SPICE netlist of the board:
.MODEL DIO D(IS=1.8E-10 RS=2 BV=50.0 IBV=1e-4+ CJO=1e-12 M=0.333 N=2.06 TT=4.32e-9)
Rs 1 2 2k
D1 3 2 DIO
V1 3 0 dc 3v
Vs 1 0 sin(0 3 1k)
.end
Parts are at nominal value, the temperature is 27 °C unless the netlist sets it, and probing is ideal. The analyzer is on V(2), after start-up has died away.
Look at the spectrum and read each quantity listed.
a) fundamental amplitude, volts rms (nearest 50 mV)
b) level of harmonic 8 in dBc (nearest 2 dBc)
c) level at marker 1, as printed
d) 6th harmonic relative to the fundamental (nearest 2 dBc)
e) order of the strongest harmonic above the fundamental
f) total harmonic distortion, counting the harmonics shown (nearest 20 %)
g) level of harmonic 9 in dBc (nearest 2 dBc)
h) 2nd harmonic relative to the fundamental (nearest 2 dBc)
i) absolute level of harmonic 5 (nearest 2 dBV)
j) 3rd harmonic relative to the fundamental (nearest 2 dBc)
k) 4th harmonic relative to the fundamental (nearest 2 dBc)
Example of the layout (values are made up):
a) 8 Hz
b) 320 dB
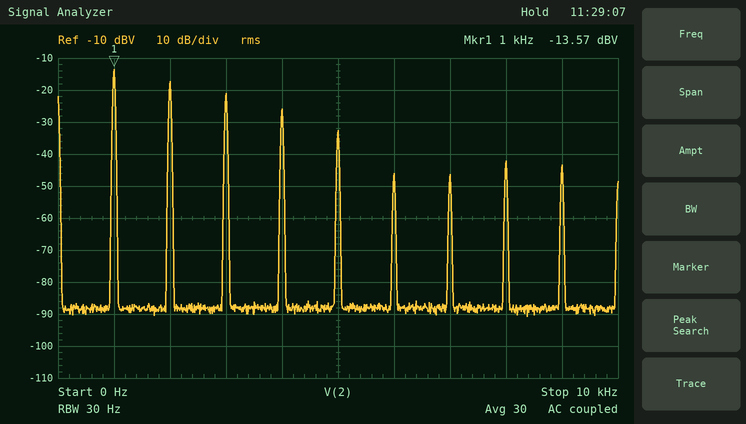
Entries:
a) 200 mV
b) -28 dBc
c) -13.57 dBV
d) -32 dBc
e) 2
f) 80 %
g) -30 dBc
h) -4 dBc
i) -32 dBV
j) -8 dBc
k) -12 dBc
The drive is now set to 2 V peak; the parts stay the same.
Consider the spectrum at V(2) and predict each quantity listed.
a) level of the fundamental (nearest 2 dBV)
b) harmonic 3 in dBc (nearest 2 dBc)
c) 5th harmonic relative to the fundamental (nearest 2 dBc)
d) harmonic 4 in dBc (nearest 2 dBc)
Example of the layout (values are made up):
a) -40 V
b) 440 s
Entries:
a) -26 dBV
b) -20 dBc
c) -34 dBc
d) -28 dBc
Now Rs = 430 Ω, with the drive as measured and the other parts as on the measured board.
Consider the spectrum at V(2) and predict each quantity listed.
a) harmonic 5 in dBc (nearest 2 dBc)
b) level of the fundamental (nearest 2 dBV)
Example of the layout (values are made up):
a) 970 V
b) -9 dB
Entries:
a) -22 dBc
b) -12 dBV
